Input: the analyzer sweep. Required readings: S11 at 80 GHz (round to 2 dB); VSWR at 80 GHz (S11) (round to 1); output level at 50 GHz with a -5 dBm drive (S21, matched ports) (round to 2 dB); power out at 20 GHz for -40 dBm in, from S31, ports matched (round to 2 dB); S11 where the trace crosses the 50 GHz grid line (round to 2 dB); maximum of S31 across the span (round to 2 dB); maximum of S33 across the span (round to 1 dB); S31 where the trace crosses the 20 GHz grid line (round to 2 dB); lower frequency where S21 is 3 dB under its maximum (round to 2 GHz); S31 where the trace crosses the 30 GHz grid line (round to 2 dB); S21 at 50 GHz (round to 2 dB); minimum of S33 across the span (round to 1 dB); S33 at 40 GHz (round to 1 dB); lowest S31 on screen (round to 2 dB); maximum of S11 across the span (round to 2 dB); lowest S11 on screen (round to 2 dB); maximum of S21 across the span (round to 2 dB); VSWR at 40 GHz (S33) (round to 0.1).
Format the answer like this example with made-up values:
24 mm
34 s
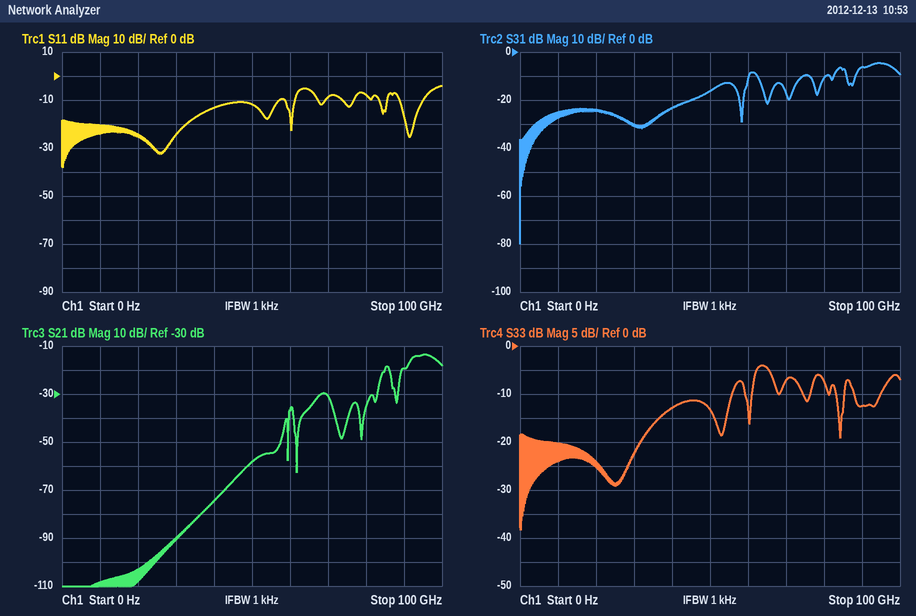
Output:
-8 dB
2
-64 dBm
-64 dBm
-12 dB
-4 dB
-4 dB
-24 dB
92 GHz
-30 dB
-58 dB
-38 dB
-13 dB
-80 dB
-4 dB
-38 dB
-14 dB
1.6
